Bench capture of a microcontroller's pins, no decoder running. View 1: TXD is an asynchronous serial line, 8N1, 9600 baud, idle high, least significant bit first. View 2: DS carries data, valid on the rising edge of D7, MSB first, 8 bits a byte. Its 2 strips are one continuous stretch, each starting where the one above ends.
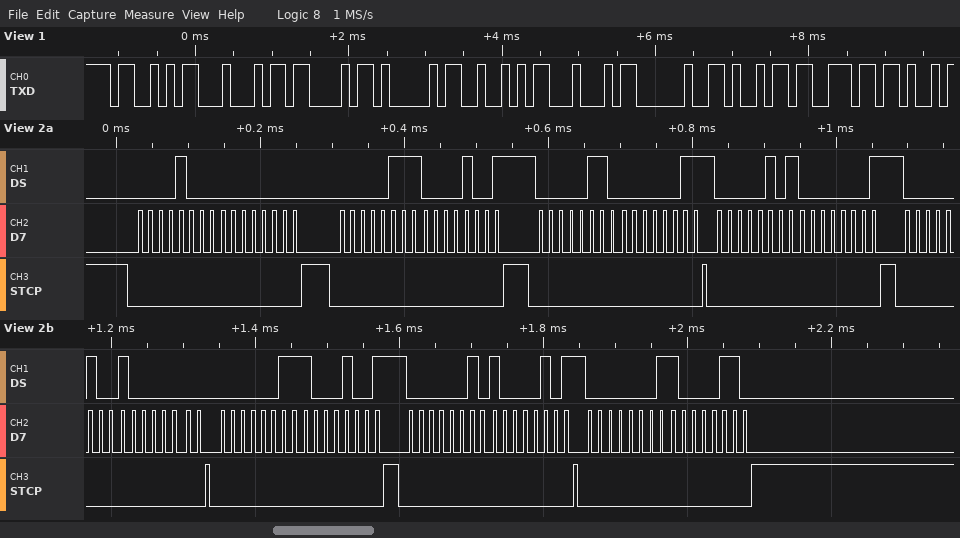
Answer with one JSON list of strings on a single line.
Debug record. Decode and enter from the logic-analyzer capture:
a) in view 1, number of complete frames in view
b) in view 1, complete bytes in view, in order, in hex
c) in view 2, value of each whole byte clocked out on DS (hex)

["9", "53 44 43 41 52 44 20 69 6E", "0x08 0x00 0x07 0x09 0x06 0x03 0x05 0x01 0x04 0x80 0x03 0x89 0x02 0x85 0x01 0x86"]
